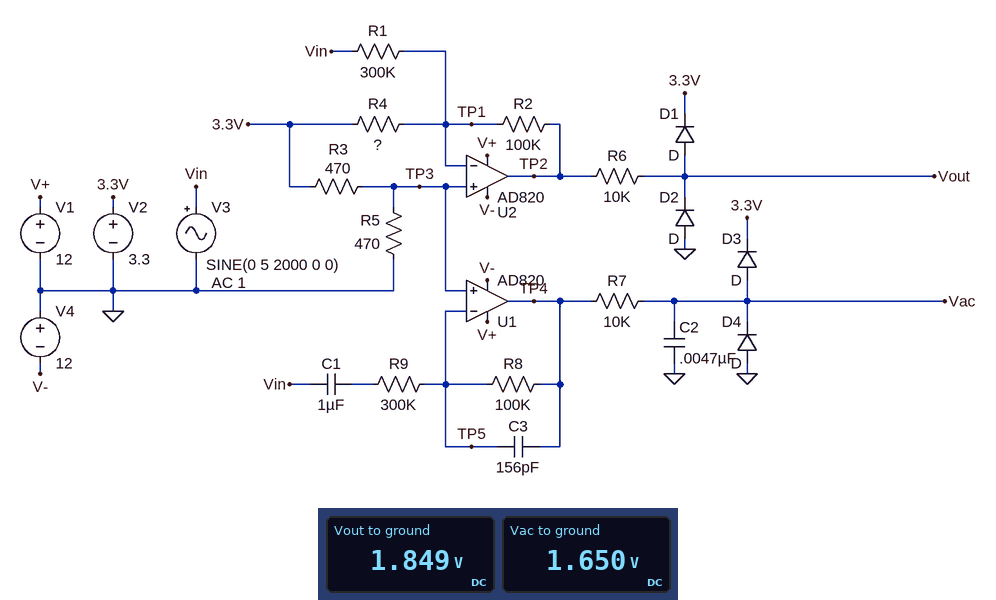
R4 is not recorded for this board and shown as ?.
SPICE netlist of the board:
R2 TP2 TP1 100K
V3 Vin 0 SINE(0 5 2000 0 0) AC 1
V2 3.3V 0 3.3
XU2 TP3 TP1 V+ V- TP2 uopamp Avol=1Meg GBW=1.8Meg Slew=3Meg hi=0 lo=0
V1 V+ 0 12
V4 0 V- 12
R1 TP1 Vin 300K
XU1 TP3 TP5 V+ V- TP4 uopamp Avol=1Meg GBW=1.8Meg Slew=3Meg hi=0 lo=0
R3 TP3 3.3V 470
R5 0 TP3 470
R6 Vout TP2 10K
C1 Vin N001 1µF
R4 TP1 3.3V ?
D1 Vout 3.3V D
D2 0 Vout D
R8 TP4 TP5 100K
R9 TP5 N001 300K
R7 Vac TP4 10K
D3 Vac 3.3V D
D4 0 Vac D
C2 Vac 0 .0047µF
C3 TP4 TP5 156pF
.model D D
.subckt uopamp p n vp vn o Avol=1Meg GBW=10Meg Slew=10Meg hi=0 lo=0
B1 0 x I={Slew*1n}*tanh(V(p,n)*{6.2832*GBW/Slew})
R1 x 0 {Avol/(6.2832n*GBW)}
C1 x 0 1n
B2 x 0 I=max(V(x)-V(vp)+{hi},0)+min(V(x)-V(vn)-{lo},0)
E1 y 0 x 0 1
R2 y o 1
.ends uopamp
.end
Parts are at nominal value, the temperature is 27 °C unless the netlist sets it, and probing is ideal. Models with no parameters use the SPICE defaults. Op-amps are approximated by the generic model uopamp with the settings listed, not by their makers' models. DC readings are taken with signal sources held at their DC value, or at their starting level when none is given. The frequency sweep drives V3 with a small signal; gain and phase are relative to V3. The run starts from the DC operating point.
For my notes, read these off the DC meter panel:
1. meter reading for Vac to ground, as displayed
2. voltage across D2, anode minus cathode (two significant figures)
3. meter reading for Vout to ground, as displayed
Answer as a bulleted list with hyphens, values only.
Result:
- 1.650 V
- -1.8 V
- 1.849 V
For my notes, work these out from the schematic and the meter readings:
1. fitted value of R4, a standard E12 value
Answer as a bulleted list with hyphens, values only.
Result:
- 470 kΩ
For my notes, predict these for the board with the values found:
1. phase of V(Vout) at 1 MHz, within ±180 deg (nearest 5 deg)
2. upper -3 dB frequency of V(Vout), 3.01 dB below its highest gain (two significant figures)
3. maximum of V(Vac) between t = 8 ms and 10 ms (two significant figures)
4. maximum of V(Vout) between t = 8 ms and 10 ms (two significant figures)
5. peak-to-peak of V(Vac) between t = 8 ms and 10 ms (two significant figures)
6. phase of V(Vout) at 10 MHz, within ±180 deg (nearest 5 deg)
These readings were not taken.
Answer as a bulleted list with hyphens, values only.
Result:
- 140 deg
- 1.2 MHz
- 3.1 V
- 3.5 V
- 2.8 V
- 95 deg
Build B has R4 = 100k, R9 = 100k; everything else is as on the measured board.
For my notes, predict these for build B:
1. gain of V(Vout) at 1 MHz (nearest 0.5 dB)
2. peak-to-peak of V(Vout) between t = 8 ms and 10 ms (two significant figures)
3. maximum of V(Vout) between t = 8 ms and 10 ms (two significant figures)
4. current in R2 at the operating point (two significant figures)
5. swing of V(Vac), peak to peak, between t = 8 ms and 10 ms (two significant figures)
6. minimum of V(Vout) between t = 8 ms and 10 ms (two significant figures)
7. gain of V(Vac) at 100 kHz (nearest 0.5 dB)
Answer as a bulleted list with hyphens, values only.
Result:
- -14.0 dB
- 2.8 V
- 2.2 V
- 11 µA
- 4.5 V
- -580 mV
- -49.5 dB
